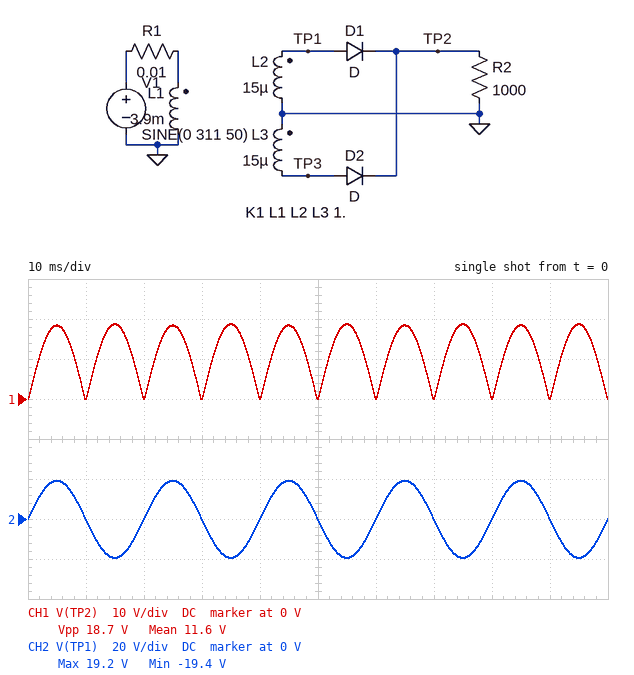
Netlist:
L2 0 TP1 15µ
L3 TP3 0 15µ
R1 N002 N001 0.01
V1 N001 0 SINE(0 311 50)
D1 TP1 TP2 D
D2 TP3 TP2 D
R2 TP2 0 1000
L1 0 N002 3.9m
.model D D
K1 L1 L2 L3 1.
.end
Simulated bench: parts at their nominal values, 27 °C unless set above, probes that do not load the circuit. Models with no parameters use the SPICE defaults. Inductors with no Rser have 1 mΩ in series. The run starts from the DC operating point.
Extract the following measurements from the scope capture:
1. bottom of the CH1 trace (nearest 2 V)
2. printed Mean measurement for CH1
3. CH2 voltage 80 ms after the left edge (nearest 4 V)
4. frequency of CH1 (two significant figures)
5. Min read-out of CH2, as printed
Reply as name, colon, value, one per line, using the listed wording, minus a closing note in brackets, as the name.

bottom of the CH1 trace: 0 V
printed Mean measurement for CH1: 11.6 V
CH2 voltage 80 ms after the left edge: 0 V
frequency of CH1: 100 Hz
Min read-out of CH2, as printed: -19.4 V
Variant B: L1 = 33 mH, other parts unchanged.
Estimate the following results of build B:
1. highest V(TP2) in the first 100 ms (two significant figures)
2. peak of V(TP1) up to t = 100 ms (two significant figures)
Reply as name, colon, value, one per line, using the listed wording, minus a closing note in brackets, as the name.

highest V(TP2) in the first 100 ms: 5.9 V
peak of V(TP1) up to t = 100 ms: 6.6 V
